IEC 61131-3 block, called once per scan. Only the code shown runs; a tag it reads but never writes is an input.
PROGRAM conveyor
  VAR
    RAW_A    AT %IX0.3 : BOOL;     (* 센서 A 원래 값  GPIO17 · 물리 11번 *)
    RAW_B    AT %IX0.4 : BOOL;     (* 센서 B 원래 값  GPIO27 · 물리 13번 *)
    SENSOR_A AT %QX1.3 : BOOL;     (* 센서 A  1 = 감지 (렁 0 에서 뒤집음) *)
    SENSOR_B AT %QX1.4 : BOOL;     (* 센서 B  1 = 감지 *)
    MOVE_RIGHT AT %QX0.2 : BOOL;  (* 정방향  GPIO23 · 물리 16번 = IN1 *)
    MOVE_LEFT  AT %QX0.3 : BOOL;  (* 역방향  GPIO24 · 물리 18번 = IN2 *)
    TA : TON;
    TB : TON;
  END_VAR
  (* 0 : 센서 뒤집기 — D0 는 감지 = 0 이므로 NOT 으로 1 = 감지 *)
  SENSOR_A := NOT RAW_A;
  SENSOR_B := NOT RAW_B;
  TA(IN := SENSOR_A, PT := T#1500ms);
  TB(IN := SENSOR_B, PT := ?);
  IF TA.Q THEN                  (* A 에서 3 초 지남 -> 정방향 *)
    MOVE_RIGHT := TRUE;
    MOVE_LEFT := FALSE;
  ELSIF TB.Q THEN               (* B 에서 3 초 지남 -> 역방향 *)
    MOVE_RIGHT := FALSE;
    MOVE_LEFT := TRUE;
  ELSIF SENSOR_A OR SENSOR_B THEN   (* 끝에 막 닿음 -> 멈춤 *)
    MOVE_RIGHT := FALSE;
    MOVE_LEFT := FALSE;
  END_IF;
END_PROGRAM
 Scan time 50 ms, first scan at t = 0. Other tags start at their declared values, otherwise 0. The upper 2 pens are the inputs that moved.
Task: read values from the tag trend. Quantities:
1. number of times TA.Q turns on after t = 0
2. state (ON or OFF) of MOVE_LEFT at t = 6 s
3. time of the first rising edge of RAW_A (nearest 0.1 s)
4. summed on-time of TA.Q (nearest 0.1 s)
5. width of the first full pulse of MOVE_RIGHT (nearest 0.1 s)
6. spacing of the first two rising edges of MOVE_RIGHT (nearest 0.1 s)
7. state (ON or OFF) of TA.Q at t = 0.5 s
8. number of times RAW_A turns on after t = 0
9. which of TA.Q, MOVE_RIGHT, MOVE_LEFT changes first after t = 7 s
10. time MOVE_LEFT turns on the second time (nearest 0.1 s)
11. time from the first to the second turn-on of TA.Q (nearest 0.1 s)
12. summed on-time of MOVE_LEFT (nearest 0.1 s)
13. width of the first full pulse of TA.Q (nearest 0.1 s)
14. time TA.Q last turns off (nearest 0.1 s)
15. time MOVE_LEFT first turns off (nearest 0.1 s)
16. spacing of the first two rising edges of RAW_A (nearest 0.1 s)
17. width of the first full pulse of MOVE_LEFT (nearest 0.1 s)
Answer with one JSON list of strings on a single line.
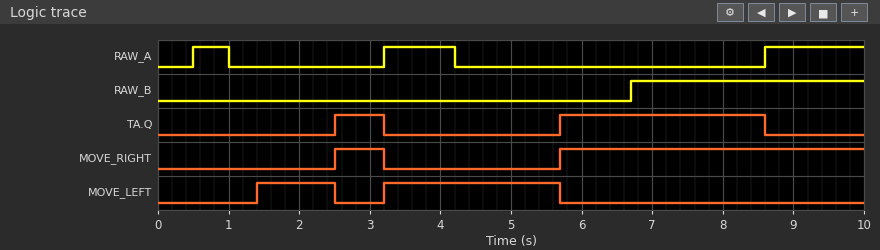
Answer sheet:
["2", "OFF", "0.5 s", "3.6 s", "0.7 s", "3.2 s", "OFF", "3", "TA.Q", "3.2 s", "3.2 s", "3.6 s", "0.7 s", "8.6 s", "2.5 s", "2.7 s", "1.1 s"]
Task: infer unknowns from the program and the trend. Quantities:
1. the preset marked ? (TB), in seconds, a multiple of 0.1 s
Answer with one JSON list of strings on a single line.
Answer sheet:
["1.4 s"]
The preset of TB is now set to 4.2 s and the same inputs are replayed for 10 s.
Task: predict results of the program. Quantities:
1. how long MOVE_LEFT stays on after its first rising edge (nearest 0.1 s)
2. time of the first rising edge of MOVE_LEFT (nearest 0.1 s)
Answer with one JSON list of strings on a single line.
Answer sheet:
["1.5 s", "4.2 s"]
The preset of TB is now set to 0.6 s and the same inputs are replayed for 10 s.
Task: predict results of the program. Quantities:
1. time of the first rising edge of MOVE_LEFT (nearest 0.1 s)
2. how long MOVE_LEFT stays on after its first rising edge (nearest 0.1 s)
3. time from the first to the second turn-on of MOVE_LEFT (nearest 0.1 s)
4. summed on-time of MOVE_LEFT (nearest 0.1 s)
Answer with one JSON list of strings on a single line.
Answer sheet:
["0.6 s", "1.9 s", "2.6 s", "4.4 s"]
